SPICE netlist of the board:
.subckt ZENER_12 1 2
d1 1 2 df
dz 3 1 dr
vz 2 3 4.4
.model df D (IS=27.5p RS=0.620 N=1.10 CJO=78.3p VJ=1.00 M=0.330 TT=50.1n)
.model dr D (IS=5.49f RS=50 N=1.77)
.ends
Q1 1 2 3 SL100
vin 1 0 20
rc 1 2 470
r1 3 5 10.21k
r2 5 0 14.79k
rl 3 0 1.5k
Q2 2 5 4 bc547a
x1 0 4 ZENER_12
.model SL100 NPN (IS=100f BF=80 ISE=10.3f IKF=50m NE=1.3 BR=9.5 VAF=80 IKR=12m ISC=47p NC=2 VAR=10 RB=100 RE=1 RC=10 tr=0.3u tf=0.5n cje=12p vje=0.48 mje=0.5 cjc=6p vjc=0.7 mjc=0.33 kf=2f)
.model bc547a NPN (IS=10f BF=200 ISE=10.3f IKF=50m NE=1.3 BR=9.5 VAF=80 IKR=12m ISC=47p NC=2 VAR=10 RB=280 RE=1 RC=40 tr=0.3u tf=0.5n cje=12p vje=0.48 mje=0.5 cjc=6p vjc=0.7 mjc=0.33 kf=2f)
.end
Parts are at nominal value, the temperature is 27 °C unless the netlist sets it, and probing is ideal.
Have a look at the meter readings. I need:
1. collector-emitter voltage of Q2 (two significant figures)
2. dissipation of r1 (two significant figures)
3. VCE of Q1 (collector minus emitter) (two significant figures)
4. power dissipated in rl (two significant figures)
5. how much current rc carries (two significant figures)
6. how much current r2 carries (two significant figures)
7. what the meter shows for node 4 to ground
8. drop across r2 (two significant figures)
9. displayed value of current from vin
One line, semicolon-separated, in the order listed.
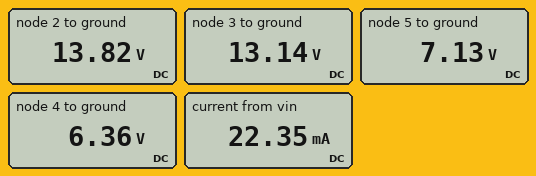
7.5 V; 3.5 mW; 6.9 V; 120 mW; 13 mA; 480 µA; 6.36 V; 7.1 V; 22.35 mA
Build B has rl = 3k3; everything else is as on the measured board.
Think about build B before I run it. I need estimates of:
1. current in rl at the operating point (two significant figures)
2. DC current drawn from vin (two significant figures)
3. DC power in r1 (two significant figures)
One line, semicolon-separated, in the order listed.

4.0 mA; 18 mA; 3.6 mW
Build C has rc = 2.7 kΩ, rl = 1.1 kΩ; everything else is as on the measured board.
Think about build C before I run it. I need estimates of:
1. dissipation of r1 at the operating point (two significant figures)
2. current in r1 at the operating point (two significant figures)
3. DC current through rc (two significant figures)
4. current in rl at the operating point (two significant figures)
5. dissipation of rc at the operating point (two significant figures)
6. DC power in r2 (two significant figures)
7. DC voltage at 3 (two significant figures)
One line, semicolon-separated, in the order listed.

2.2 mW; 460 µA; 3.0 mA; 10 mA; 25 mW; 2.8 mW; 11 V
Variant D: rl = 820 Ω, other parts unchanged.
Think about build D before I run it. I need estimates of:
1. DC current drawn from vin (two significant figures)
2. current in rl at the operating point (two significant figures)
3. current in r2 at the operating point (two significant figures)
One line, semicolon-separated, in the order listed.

29 mA; 16 mA; 480 µA
